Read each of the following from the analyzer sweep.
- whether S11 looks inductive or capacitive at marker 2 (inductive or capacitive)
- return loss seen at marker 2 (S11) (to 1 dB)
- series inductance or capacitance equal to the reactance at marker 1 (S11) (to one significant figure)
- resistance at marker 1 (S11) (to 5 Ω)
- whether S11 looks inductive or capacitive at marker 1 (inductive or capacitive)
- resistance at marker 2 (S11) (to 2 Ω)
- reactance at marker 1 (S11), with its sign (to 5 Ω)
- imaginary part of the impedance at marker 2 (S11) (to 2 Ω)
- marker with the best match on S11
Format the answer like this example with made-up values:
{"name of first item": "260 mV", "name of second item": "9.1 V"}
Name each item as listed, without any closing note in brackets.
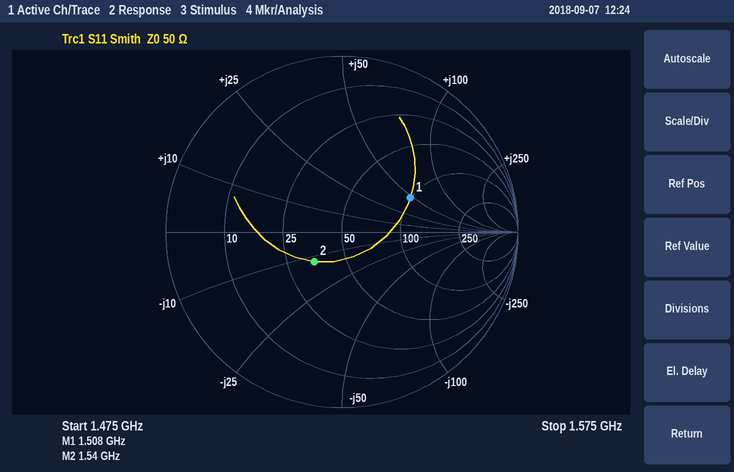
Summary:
{"whether S11 looks inductive or capacitive at marker 2": "capacitive", "return loss seen at marker 2 (S11)": "13 dB", "series inductance or capacitance equal to the reactance at marker 1 (S11)": "5 nH", "resistance at marker 1 (S11)": "100 Ω", "whether S11 looks inductive or capacitive at marker 1": "inductive", "resistance at marker 2 (S11)": "34 Ω", "reactance at marker 1 (S11), with its sign": "+45 Ω", "imaginary part of the impedance at marker 2 (S11)": "-12 Ω", "marker with the best match on S11": "marker 2"}
